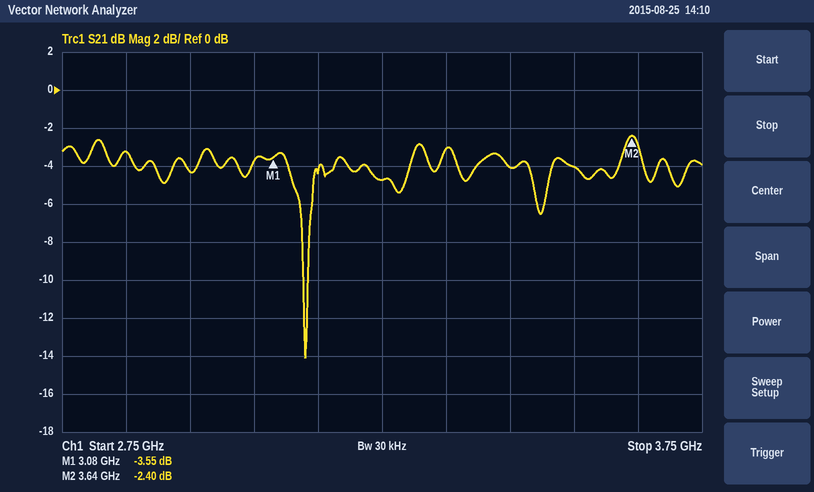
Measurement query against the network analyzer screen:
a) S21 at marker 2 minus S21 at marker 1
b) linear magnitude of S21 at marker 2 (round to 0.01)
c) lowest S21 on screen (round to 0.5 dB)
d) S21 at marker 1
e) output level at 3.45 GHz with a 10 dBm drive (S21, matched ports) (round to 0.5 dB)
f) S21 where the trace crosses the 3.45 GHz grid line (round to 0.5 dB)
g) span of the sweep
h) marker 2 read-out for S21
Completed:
1.15 dB
0.76
-14.0 dB
-3.55 dB
6.0 dBm
-4.0 dB
1 GHz
-2.40 dB
